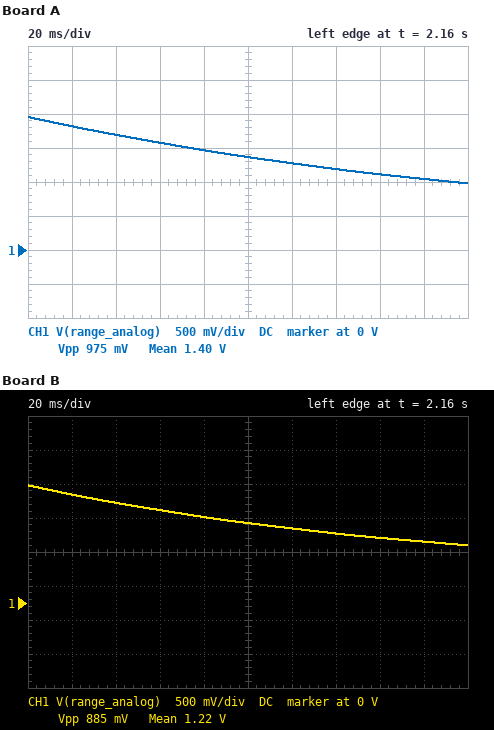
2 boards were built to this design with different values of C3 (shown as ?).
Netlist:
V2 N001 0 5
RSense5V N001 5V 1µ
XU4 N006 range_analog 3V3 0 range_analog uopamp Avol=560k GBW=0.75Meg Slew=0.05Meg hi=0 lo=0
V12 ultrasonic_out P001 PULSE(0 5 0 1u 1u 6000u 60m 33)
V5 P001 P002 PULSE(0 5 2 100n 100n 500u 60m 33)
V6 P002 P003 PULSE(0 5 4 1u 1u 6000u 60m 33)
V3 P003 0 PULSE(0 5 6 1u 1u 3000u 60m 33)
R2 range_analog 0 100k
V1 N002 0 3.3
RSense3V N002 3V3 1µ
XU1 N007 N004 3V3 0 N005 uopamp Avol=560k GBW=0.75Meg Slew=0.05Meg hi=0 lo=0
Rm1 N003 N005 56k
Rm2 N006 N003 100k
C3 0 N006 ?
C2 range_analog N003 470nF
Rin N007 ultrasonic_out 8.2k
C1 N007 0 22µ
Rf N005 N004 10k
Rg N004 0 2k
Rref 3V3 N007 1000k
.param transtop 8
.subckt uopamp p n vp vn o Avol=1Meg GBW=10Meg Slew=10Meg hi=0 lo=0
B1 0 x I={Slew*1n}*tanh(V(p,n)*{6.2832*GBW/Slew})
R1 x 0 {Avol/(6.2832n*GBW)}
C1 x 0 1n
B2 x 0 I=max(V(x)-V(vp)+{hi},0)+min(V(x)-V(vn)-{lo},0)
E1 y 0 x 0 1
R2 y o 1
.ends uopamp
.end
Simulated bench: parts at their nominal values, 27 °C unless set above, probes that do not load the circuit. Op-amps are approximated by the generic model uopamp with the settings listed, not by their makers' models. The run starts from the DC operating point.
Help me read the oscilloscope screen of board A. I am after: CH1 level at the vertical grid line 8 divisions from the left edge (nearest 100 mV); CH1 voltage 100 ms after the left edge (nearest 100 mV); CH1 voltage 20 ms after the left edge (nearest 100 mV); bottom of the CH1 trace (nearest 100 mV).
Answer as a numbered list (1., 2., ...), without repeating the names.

1. 1.1 V
2. 1.4 V
3. 1.8 V
4. 1.0 V
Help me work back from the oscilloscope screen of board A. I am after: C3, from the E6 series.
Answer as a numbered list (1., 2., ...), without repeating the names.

1. 680 nF
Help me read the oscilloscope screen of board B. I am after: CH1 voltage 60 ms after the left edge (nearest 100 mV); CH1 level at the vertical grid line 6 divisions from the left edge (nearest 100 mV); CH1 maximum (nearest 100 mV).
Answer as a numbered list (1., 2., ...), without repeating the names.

1. 1.4 V
2. 1.1 V
3. 1.7 V
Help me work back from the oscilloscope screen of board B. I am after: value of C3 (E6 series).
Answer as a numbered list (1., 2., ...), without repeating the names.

1. 470 nF
